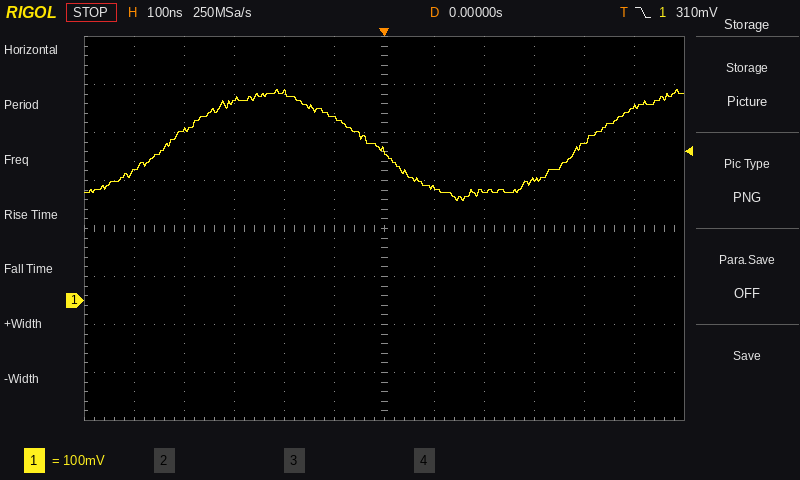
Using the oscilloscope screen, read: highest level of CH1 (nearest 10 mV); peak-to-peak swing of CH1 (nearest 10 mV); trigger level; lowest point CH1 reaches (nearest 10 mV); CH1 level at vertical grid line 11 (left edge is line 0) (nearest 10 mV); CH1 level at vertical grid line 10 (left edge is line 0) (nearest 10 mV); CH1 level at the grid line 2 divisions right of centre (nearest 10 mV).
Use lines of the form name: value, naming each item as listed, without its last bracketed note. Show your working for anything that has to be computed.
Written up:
highest level of CH1: 440 mV
peak-to-peak swing of CH1: 440 mV − (210 mV) = 230 mV
trigger level: 310 mV
lowest point CH1 reaches: 210 mV
CH1 level at vertical grid line 11 (left edge is line 0): 400 mV
CH1 level at vertical grid line 10 (left edge is line 0): 330 mV
CH1 level at the grid line 2 divisions right of centre: 230 mV
